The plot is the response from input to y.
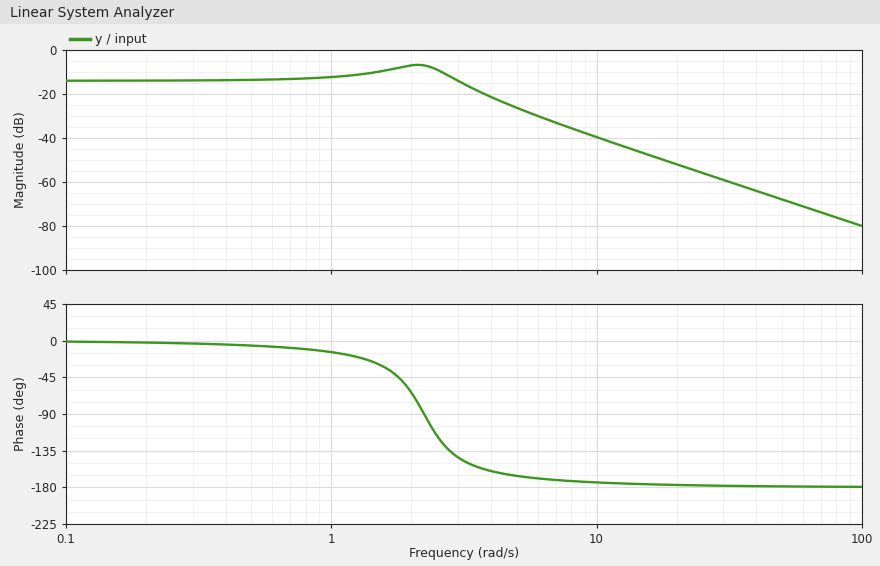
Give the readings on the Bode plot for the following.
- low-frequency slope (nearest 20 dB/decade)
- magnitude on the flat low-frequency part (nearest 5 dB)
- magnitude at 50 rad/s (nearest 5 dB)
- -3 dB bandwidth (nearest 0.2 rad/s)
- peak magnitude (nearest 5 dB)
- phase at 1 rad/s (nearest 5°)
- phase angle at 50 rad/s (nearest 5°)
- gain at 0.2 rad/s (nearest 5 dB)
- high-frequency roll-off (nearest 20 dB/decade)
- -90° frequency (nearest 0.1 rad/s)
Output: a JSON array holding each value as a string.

["0 dB/decade", "-15 dB", "-70 dB", "3.4 rad/s", "-5 dB", "-15°", "-180°", "-15 dB", "-40 dB/decade", "2.2 rad/s"]
